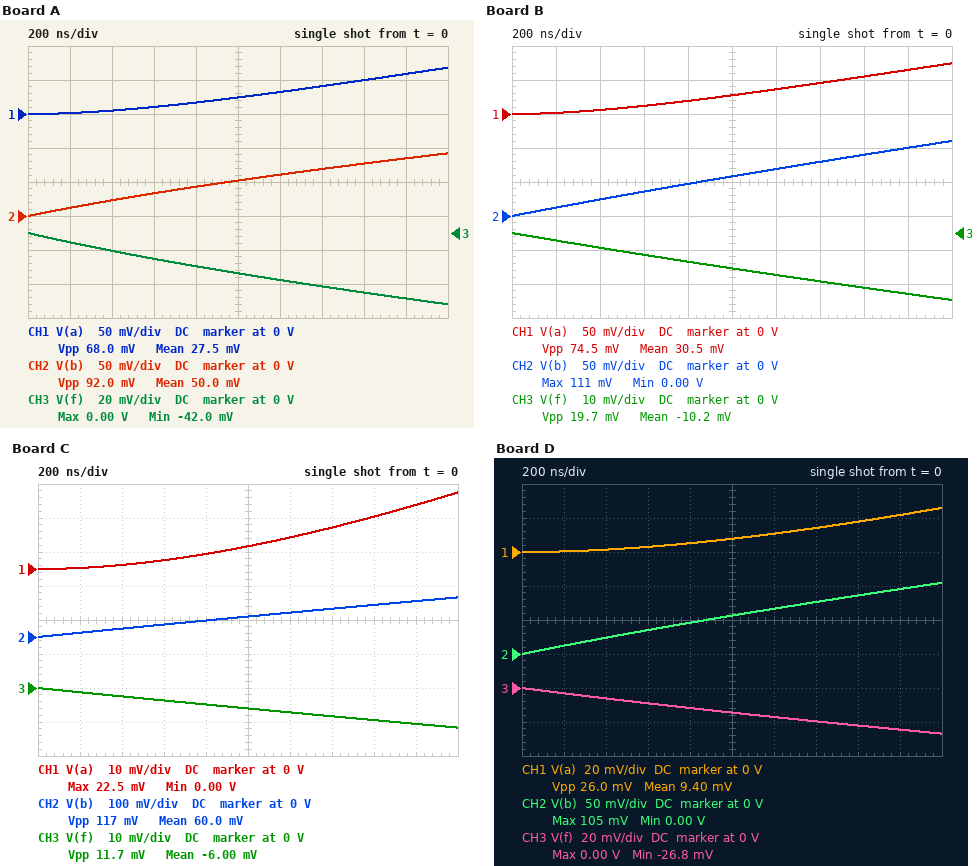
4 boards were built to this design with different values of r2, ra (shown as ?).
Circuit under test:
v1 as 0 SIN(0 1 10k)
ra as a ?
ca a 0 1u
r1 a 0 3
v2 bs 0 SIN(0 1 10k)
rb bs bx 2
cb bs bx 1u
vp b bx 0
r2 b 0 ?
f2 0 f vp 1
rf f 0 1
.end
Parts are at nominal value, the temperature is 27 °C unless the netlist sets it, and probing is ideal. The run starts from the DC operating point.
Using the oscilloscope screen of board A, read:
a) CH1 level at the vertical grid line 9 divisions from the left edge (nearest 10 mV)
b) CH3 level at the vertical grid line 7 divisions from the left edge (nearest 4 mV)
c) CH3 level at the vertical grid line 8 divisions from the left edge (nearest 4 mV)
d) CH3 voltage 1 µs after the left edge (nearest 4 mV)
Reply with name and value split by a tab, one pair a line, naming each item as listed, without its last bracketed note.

CH1 level at the vertical grid line 9 divisions from the left edge	60 mV
CH3 level at the vertical grid line 7 divisions from the left edge	-32 mV
CH3 level at the vertical grid line 8 divisions from the left edge	-36 mV
CH3 voltage 1 µs after the left edge	-24 mV
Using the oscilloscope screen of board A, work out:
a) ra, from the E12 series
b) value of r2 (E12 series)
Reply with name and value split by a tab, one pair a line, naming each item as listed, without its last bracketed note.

ra, from the E12 series	0.82 Ω
value of r2	2.2 Ω
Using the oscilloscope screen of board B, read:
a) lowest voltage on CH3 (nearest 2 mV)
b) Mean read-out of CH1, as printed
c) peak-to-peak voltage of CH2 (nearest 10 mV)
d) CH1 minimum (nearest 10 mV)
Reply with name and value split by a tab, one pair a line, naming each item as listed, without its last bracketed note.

lowest voltage on CH3	-20 mV
Mean read-out of CH1, as printed	30.5 mV
peak-to-peak voltage of CH2	110 mV
CH1 minimum	0 V
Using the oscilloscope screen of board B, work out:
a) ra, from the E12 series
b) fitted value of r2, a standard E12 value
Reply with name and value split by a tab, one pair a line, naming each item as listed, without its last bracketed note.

ra, from the E12 series	0.68 Ω
fitted value of r2, a standard E12 value	5.6 Ω
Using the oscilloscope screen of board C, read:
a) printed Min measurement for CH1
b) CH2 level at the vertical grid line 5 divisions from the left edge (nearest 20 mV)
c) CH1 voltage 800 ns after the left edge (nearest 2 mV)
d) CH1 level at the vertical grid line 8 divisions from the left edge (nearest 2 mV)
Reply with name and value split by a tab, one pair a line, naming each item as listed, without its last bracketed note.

printed Min measurement for CH1	0.00 V
CH2 level at the vertical grid line 5 divisions from the left edge	60 mV
CH1 voltage 800 ns after the left edge	4 mV
CH1 level at the vertical grid line 8 divisions from the left edge	16 mV
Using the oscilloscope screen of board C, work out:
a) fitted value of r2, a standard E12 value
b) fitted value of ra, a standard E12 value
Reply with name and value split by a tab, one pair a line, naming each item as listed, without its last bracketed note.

fitted value of r2, a standard E12 value	10 Ω
fitted value of ra, a standard E12 value	3.9 Ω
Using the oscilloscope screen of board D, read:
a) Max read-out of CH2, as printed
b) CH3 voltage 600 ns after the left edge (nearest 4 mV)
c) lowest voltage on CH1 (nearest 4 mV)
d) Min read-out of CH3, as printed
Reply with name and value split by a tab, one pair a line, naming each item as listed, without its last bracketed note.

Max read-out of CH2, as printed	105 mV
CH3 voltage 600 ns after the left edge	-8 mV
lowest voltage on CH1	0 V
Min read-out of CH3, as printed	-26.8 mV
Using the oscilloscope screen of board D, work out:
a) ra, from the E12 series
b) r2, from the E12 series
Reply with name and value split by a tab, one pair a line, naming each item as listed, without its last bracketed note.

ra, from the E12 series	3.3 Ω
r2, from the E12 series	3.9 Ω
